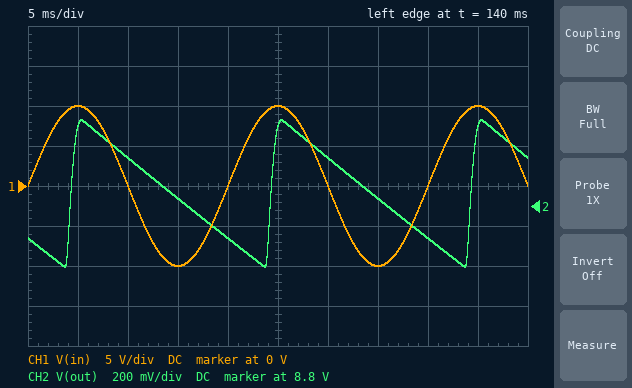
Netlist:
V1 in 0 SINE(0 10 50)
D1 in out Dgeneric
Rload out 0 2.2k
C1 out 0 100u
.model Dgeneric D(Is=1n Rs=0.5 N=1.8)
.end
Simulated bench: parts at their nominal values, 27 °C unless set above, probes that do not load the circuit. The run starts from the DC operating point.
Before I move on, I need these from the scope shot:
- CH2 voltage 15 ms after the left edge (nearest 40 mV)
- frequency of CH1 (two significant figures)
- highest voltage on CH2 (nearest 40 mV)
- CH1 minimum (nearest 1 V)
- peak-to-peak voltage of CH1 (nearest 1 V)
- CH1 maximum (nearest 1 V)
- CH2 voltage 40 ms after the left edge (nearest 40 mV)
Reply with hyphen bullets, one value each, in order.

- 8.84 V
- 50 Hz
- 9.24 V
- -10 V
- 20 V
- 10 V
- 8.64 V
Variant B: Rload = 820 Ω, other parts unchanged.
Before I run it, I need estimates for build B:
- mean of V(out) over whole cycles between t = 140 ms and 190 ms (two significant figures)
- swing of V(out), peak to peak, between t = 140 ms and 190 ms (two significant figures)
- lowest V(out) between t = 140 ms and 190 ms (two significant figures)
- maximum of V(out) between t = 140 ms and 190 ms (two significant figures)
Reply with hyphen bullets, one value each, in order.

- 8.3 V
- 1.8 V
- 7.4 V
- 9.2 V
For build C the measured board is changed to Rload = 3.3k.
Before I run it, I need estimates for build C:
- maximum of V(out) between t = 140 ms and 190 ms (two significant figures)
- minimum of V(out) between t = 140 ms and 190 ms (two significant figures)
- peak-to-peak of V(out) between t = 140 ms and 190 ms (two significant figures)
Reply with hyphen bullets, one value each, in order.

- 9.2 V
- 8.7 V
- 500 mV
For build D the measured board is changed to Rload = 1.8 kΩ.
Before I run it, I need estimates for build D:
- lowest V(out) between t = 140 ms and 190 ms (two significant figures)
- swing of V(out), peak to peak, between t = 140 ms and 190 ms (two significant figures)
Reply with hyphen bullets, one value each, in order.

- 8.3 V
- 880 mV
